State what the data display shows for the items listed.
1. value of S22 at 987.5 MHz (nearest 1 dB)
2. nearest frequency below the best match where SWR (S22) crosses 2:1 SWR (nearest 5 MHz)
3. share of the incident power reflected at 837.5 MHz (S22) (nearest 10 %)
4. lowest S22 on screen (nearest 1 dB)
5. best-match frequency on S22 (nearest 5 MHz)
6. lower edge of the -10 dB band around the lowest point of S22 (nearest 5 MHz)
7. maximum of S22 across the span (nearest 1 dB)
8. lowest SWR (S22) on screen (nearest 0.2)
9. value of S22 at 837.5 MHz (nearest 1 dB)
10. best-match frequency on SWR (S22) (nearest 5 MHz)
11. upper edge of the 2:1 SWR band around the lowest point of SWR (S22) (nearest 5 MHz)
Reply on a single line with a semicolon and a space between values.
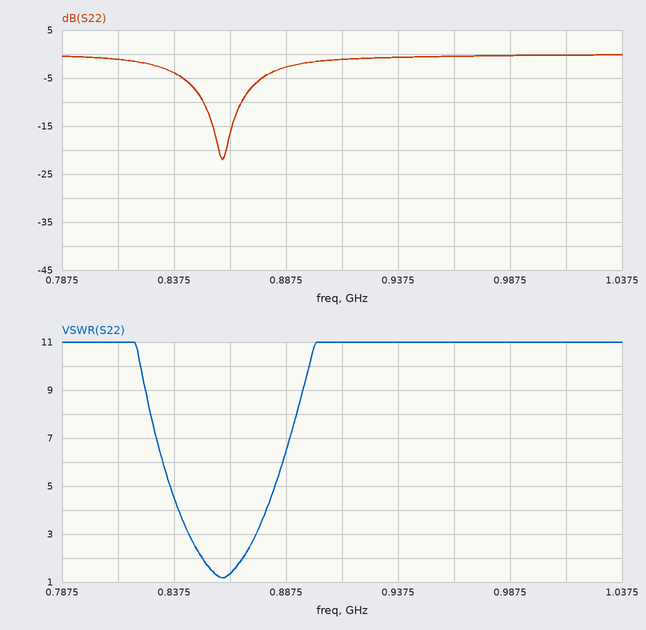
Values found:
0 dB; 850 MHz; 40 %; -22 dB; 860 MHz; 850 MHz; 0 dB; 1.2; -4 dB; 860 MHz; 870 MHz
